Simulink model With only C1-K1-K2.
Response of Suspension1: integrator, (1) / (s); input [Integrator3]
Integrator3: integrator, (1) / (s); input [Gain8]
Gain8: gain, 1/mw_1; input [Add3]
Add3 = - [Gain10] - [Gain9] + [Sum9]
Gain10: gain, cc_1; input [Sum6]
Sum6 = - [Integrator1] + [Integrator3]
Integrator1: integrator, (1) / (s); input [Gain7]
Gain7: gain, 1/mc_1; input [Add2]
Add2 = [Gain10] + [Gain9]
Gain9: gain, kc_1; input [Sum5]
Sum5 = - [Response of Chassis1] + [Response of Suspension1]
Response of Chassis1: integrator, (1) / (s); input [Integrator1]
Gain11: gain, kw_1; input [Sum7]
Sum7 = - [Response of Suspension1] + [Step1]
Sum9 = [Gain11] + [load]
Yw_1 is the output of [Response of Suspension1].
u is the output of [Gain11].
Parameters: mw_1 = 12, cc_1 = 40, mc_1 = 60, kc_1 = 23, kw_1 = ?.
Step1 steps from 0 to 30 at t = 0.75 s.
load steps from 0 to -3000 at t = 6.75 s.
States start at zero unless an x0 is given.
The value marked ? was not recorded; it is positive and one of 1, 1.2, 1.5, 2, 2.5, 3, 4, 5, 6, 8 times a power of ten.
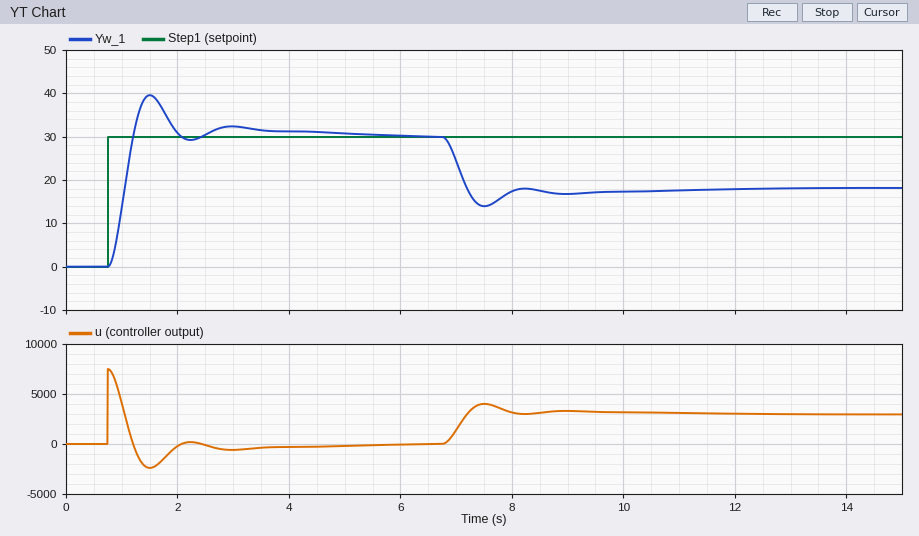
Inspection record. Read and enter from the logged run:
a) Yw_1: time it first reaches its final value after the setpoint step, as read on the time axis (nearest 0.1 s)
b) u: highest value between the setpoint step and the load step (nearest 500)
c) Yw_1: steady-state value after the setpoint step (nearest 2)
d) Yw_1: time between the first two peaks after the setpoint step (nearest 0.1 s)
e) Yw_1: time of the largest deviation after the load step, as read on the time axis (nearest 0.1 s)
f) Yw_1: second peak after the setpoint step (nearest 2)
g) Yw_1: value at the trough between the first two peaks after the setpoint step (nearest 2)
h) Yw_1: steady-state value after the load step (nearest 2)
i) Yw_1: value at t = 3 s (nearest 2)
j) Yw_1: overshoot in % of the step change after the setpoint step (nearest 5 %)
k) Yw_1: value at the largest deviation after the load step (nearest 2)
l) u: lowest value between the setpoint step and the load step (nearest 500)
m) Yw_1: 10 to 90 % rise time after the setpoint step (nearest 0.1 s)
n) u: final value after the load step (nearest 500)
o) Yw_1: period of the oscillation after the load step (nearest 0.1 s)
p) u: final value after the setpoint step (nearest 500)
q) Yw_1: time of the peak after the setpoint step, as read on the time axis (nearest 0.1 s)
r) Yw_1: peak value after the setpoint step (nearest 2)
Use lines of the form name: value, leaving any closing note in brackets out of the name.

Yw_1: time it first reaches its final value after the setpoint step, as read on the time axis: 1.2 s
u: highest value between the setpoint step and the load step: 7500
Yw_1: steady-state value after the setpoint step: 30
Yw_1: time between the first two peaks after the setpoint step: 1.5 s
Yw_1: time of the largest deviation after the load step, as read on the time axis: 7.5 s
Yw_1: second peak after the setpoint step: 32
Yw_1: value at the trough between the first two peaks after the setpoint step: 30
Yw_1: steady-state value after the load step: 18
Yw_1: value at t = 3 s: 32
Yw_1: overshoot in % of the step change after the setpoint step: 30 %
Yw_1: value at the largest deviation after the load step: 14
u: lowest value between the setpoint step and the load step: -2500
Yw_1: 10 to 90 % rise time after the setpoint step: 0.3 s
u: final value after the load step: 3000
Yw_1: period of the oscillation after the load step: 1.5 s
u: final value after the setpoint step: 0
Yw_1: time of the peak after the setpoint step, as read on the time axis: 1.5 s
Yw_1: peak value after the setpoint step: 40
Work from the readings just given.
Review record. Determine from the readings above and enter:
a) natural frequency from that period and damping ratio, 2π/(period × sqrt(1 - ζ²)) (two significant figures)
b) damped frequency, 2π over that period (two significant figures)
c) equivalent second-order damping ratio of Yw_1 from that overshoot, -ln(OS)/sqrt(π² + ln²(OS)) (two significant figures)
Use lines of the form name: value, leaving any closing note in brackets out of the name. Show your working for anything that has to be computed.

natural frequency from that period and damping ratio, 2π/(period × sqrt(1 - ζ²)): 2π / (1.5 × sqrt(1 - 0.36²)) = 4.5 rad/s
damped frequency, 2π over that period: 2π / 1.5 = 4.2 rad/s
equivalent second-order damping ratio of Yw_1 from that overshoot, -ln(OS)/sqrt(π² + ln²(OS)): ln(0.3) = -1.204; 1.204 / sqrt(9.870 + 1.450) = 0.36
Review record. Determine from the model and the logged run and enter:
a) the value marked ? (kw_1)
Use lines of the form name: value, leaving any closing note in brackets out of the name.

the value marked ?: 250
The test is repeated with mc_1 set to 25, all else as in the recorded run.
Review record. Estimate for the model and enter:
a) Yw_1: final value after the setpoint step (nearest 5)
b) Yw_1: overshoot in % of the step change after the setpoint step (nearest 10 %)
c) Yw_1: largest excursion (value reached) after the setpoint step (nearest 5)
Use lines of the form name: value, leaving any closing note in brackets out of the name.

Yw_1: final value after the setpoint step: 30
Yw_1: overshoot in % of the step change after the setpoint step: 50 %
Yw_1: largest excursion (value reached) after the setpoint step: 45
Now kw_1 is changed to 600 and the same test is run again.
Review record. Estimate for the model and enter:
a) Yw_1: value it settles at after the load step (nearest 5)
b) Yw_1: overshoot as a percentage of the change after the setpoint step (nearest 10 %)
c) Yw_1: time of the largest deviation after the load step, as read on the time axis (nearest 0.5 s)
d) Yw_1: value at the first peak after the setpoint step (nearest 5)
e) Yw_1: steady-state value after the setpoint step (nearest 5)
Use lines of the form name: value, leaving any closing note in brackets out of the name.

Yw_1: value it settles at after the load step: 25
Yw_1: overshoot as a percentage of the change after the setpoint step: 50 %
Yw_1: time of the largest deviation after the load step, as read on the time axis: 7.0 s
Yw_1: value at the first peak after the setpoint step: 45
Yw_1: steady-state value after the setpoint step: 30
